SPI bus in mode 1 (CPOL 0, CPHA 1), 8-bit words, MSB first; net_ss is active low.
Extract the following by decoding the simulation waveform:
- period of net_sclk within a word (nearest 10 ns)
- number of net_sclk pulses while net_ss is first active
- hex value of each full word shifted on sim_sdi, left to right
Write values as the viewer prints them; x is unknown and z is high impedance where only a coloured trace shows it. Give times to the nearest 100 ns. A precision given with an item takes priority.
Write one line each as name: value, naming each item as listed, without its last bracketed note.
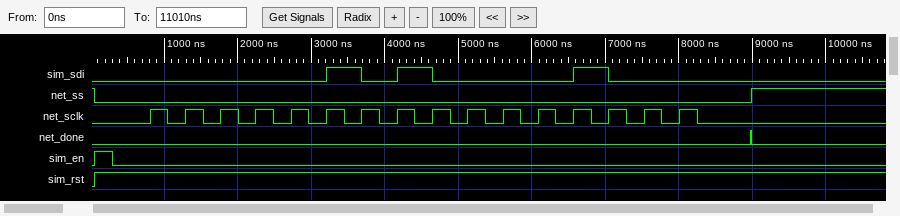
period of net_sclk within a word: 480 ns
number of net_sclk pulses while net_ss is first active: 16
hex value of each full word shifted on sim_sdi, left to right: 05, 08
